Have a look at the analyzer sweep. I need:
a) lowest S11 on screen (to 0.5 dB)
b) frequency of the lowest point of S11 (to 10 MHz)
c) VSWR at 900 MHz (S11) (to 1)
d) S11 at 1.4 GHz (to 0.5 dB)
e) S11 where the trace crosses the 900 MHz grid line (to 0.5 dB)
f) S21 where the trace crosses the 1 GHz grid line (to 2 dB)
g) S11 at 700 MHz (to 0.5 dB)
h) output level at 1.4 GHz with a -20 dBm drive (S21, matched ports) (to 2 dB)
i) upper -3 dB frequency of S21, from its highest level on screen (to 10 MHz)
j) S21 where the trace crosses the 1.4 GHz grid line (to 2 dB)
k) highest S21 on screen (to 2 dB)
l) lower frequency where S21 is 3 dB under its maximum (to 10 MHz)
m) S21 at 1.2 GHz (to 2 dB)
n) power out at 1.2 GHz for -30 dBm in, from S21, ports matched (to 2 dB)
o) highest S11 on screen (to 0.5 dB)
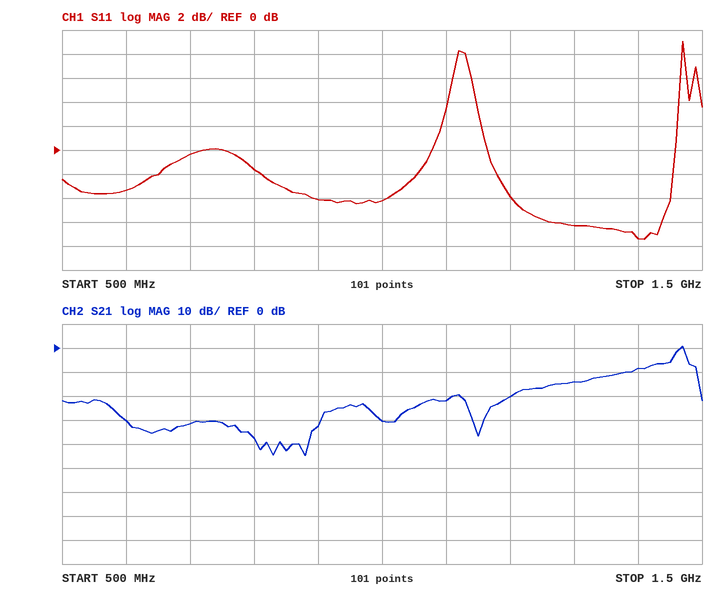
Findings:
-7.5 dB
1.41 GHz
4
-7.5 dB
-4.0 dB
-30 dB
-0.5 dB
-28 dBm
1.47 GHz
-8 dB
0 dB
1.46 GHz
-20 dB
-50 dBm
9.0 dB
